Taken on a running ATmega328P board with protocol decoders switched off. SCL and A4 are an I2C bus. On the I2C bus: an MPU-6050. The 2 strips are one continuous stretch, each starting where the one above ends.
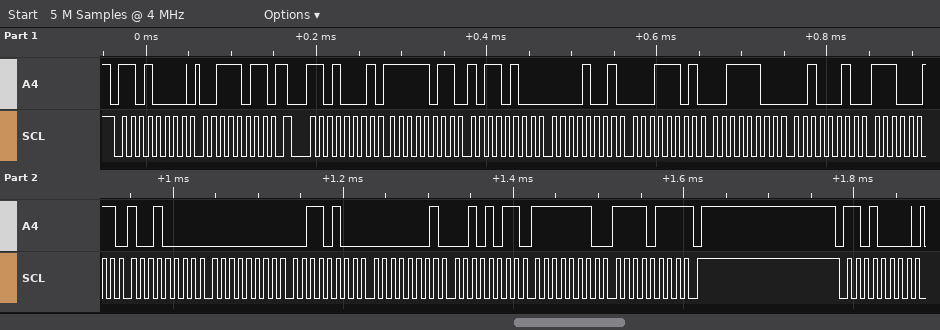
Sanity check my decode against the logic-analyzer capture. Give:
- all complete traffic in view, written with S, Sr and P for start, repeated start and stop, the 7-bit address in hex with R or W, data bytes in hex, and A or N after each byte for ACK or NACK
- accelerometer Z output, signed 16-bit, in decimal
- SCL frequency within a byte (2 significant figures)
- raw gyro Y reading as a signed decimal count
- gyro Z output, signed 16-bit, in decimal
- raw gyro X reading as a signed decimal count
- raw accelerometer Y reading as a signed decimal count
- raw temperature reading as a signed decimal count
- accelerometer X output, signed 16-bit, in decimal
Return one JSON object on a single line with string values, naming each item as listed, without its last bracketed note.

{"all complete traffic in view, written with S, Sr and P for start, repeated start and stop, the 7-bit address in hex with R or W, data bytes in hex, and A or N after each byte for ACK or NACK": "S 68W A 3B A Sr 68R A FB A B4 A 09 A 1D A 3C A 22 A E3 A 90 A 00 A 34 A 01 A 2B A FE A F7 N P S 68W A", "accelerometer Z output, signed 16-bit, in decimal": "15394", "SCL frequency within a byte": "100 kHz", "raw gyro Y reading as a signed decimal count": "299", "gyro Z output, signed 16-bit, in decimal": "-265", "raw gyro X reading as a signed decimal count": "52", "raw accelerometer Y reading as a signed decimal count": "2333", "raw temperature reading as a signed decimal count": "-7280", "accelerometer X output, signed 16-bit, in decimal": "-1100"}
